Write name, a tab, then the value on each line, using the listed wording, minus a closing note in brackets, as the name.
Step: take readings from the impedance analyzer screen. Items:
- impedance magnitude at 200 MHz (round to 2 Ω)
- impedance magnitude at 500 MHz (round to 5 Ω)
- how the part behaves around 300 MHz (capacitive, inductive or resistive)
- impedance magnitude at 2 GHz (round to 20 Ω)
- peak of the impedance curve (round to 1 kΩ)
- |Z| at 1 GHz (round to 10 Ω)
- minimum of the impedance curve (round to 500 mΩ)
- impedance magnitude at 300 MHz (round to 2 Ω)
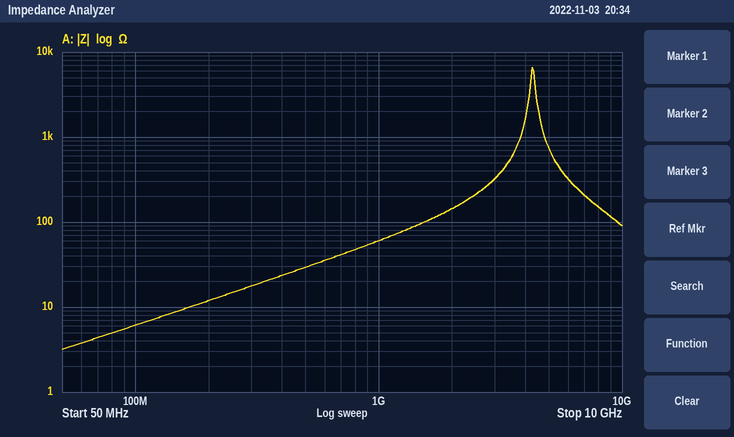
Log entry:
impedance magnitude at 200 MHz	12 Ω
impedance magnitude at 500 MHz	30 Ω
how the part behaves around 300 MHz	inductive
impedance magnitude at 2 GHz	140 Ω
peak of the impedance curve	7 kΩ
|Z| at 1 GHz	60 Ω
minimum of the impedance curve	3.0 Ω
impedance magnitude at 300 MHz	18 Ω
